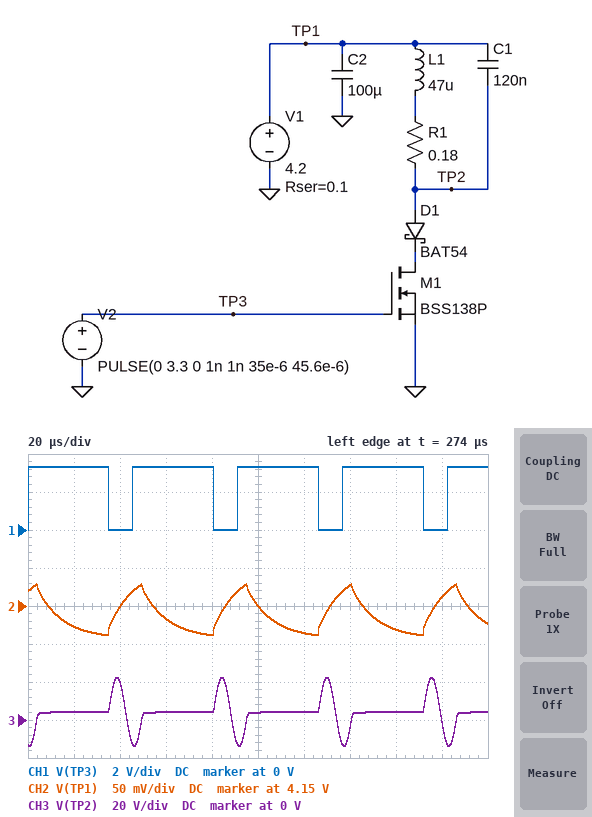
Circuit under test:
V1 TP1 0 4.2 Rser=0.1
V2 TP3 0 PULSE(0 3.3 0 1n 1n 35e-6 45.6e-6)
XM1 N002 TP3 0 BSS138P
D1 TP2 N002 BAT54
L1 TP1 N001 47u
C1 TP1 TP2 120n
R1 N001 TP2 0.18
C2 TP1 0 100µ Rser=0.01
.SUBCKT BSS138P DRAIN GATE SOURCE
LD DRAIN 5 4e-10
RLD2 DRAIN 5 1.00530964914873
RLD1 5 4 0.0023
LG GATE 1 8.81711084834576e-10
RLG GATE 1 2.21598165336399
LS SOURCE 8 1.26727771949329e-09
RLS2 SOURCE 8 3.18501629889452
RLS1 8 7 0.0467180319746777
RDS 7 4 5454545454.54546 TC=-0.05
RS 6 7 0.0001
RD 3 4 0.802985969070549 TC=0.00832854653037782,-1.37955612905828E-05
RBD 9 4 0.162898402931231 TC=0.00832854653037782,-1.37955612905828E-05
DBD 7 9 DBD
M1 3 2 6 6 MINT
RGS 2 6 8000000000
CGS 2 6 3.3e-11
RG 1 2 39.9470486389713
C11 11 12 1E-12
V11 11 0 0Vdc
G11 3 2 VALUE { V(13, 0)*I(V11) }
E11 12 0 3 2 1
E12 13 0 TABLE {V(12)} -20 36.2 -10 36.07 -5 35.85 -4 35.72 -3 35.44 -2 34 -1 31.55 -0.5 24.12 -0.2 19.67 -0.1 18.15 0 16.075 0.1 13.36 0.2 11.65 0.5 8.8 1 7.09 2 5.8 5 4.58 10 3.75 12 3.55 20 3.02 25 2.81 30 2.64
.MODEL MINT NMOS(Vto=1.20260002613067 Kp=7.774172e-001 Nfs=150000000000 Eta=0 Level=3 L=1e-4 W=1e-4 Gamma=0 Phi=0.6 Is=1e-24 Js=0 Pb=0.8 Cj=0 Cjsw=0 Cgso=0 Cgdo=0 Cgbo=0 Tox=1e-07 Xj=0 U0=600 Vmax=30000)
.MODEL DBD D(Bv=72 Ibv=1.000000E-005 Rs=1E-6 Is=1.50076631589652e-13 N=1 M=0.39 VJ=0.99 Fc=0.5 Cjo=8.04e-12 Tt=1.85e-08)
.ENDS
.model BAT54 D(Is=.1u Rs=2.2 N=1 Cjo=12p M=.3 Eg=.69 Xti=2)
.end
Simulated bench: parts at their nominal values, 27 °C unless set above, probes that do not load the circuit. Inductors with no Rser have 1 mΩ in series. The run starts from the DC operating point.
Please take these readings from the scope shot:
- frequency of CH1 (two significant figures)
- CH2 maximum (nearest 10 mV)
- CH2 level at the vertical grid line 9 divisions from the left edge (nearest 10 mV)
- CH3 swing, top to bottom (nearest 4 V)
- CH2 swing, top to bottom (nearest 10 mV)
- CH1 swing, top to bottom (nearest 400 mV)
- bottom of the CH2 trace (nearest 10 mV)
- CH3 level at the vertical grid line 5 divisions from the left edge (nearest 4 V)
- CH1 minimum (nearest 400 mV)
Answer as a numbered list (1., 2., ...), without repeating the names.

1. 22 kHz
2. 4.18 V
3. 4.16 V
4. 36 V
5. 70 mV
6. 3.2 V
7. 4.11 V
8. 4 V
9. 0 V
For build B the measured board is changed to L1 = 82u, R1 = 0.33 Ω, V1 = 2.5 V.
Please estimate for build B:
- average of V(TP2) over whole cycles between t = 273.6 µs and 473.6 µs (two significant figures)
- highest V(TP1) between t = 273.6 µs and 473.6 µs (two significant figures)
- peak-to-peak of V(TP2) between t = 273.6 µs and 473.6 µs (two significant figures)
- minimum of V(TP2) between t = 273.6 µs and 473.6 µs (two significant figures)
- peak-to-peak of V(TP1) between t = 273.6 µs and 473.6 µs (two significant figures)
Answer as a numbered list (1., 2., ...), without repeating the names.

1. 2.4 V
2. 2.5 V
3. 26 V
4. -10 V
5. 39 mV
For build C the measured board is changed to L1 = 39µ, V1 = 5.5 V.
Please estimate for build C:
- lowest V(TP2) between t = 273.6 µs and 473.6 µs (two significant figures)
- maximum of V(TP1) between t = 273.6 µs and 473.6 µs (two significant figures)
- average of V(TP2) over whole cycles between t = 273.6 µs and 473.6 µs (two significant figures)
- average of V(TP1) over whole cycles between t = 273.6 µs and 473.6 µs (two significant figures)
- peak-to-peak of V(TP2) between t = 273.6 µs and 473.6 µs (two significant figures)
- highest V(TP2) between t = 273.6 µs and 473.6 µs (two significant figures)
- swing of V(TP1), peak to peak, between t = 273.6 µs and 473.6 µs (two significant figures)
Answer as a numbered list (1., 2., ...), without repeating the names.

1. -16 V
2. 5.5 V
3. 5.3 V
4. 5.4 V
5. 43 V
6. 27 V
7. 85 mV
